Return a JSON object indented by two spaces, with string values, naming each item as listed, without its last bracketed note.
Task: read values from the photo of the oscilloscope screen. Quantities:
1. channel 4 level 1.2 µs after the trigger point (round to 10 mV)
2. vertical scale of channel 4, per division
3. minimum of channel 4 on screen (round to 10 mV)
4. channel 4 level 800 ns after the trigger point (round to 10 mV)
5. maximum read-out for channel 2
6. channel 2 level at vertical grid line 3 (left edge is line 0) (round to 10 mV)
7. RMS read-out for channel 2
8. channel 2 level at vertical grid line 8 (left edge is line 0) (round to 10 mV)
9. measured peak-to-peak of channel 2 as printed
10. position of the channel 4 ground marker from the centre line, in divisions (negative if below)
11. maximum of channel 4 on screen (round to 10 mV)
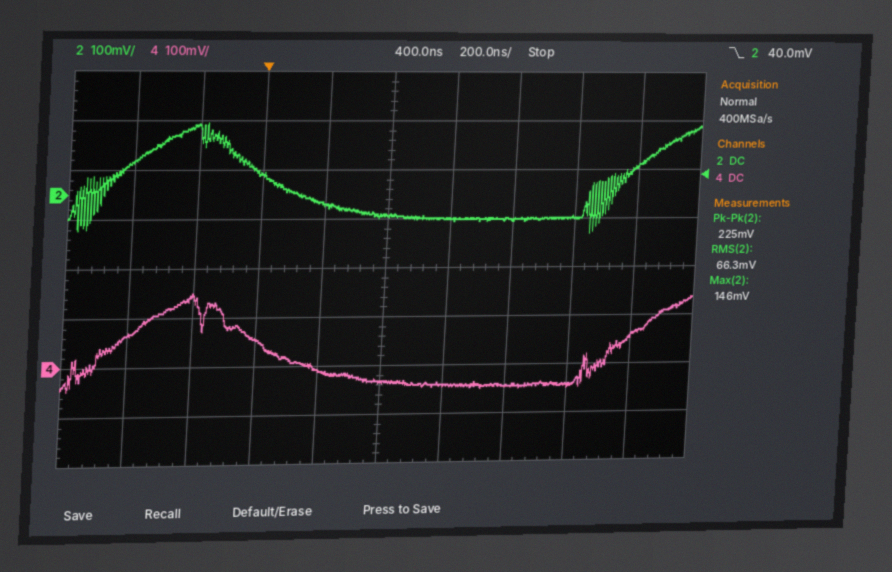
{
  "channel 4 level 1.2 µs after the trigger point": "60 mV",
  "vertical scale of channel 4, per division": "100 mV",
  "minimum of channel 4 on screen": "-50 mV",
  "channel 4 level 800 ns after the trigger point": "-40 mV",
  "maximum read-out for channel 2": "146 mV",
  "channel 2 level at vertical grid line 3 (left edge is line 0)": "40 mV",
  "RMS read-out for channel 2": "66.3 mV",
  "channel 2 level at vertical grid line 8 (left edge is line 0)": "-50 mV",
  "measured peak-to-peak of channel 2 as printed": "225 mV",
  "position of the channel 4 ground marker from the centre line, in divisions": "-2.0 div",
  "maximum of channel 4 on screen": "150 mV"
}
